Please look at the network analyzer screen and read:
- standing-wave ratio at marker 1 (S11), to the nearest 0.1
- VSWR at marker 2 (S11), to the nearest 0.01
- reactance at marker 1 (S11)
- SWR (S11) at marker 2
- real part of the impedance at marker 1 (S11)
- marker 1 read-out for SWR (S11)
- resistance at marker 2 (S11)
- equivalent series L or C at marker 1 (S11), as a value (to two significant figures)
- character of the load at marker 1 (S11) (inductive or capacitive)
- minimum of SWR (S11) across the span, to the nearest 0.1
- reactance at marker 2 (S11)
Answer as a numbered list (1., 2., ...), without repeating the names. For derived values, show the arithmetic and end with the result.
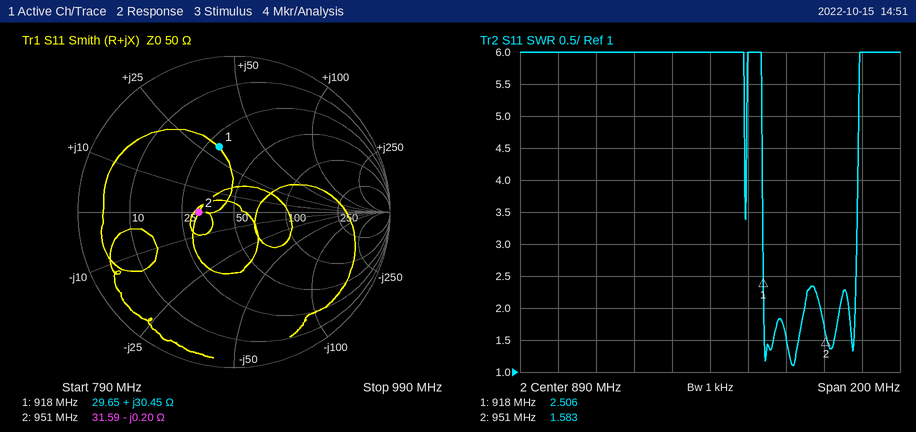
1. 2.5
2. 1.58
3. +30.45 Ω
4. 1.583
5. 29.65 Ω
6. 2.506
7. 31.59 Ω
8. L = 30.45 Ω/(2π × 918 MHz) ≈ 5.3 nH
9. inductive
10. 1.1
11. -0.20 Ω
